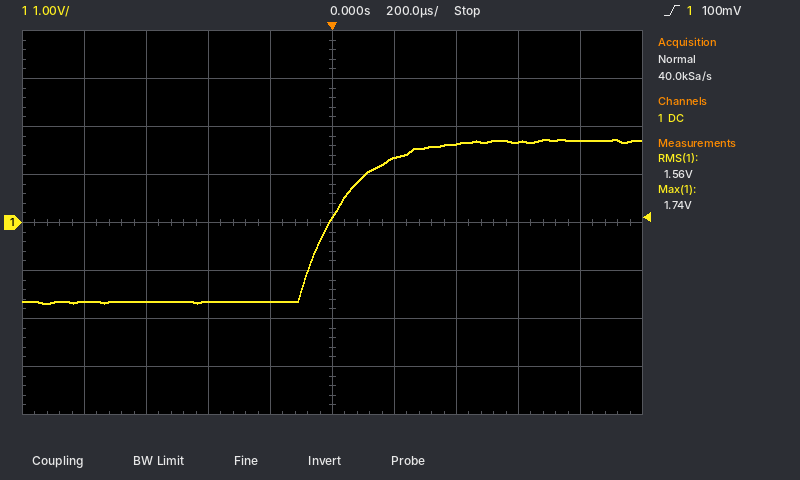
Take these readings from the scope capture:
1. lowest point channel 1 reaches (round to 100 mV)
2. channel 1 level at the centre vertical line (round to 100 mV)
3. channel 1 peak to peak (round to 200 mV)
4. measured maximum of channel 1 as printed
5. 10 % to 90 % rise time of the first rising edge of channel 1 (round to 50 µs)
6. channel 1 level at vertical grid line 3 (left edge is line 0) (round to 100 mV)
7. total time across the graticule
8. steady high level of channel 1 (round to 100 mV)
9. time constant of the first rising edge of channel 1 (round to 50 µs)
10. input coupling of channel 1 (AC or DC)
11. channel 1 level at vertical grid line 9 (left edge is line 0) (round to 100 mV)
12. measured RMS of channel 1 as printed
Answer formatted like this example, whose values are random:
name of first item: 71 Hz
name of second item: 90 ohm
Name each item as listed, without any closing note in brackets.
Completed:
lowest point channel 1 reaches: -1.7 V
channel 1 level at the centre vertical line: 100 mV
channel 1 peak to peak: 3.4 V
measured maximum of channel 1 as printed: 1.74 V
10 % to 90 % rise time of the first rising edge of channel 1: 300 µs
channel 1 level at vertical grid line 3 (left edge is line 0): -1.6 V
total time across the graticule: 2 ms
steady high level of channel 1: 1.7 V
time constant of the first rising edge of channel 1: 150 µs
input coupling of channel 1: DC
channel 1 level at vertical grid line 9 (left edge is line 0): 1.7 V
measured RMS of channel 1 as printed: 1.56 V
